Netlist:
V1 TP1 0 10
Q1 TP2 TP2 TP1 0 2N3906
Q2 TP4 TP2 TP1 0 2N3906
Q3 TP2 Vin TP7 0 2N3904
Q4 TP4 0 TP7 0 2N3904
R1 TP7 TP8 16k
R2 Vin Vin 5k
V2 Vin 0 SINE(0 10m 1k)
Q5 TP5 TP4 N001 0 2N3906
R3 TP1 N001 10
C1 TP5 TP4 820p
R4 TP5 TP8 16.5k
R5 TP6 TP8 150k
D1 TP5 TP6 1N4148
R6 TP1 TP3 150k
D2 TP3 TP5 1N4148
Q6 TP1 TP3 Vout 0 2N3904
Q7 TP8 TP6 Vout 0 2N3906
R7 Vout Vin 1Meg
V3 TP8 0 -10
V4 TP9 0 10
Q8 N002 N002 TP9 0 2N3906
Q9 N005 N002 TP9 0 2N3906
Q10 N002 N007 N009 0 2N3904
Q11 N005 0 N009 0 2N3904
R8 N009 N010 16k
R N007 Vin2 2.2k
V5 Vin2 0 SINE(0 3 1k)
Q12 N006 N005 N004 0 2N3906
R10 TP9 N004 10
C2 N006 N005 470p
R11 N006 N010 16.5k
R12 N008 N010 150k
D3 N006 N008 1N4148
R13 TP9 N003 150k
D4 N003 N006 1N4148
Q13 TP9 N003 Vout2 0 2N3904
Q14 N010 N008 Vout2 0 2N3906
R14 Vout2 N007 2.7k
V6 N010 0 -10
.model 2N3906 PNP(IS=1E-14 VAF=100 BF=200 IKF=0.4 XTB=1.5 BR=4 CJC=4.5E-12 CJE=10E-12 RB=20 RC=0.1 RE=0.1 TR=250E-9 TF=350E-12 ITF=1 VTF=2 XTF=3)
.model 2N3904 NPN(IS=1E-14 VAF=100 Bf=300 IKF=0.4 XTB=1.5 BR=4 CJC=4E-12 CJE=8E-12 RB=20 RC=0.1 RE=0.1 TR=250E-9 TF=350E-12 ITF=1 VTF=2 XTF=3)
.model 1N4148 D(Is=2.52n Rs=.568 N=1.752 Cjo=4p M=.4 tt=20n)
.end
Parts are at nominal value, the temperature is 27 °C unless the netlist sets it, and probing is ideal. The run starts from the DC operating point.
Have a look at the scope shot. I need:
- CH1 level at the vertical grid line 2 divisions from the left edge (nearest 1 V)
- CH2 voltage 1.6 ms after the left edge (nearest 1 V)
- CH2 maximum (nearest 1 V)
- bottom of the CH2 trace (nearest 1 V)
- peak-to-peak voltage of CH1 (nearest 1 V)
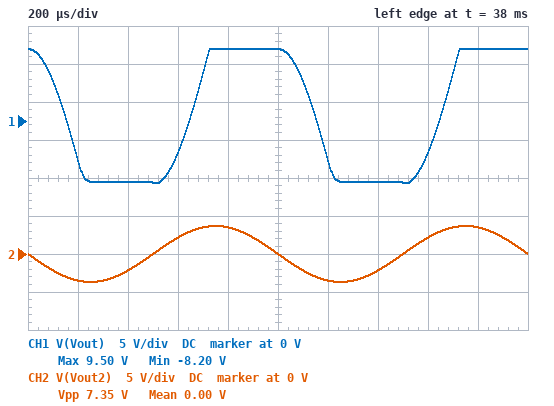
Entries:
-8 V
2 V
4 V
-4 V
18 V
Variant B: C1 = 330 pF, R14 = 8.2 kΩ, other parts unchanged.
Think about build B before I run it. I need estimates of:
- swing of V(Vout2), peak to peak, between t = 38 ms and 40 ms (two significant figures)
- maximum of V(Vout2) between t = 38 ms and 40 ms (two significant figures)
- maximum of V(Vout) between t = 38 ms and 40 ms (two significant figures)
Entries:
17 V
8.9 V
9.5 V
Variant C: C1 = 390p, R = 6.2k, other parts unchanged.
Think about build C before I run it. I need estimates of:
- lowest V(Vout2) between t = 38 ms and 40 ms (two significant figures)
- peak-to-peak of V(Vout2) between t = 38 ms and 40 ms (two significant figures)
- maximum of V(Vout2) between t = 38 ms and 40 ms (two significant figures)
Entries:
-1.3 V
2.6 V
1.3 V
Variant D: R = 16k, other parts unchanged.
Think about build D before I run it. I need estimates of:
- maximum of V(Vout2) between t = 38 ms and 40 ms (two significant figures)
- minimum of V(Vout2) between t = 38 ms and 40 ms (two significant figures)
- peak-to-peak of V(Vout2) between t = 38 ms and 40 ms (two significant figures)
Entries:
510 mV
-500 mV
1.0 V
